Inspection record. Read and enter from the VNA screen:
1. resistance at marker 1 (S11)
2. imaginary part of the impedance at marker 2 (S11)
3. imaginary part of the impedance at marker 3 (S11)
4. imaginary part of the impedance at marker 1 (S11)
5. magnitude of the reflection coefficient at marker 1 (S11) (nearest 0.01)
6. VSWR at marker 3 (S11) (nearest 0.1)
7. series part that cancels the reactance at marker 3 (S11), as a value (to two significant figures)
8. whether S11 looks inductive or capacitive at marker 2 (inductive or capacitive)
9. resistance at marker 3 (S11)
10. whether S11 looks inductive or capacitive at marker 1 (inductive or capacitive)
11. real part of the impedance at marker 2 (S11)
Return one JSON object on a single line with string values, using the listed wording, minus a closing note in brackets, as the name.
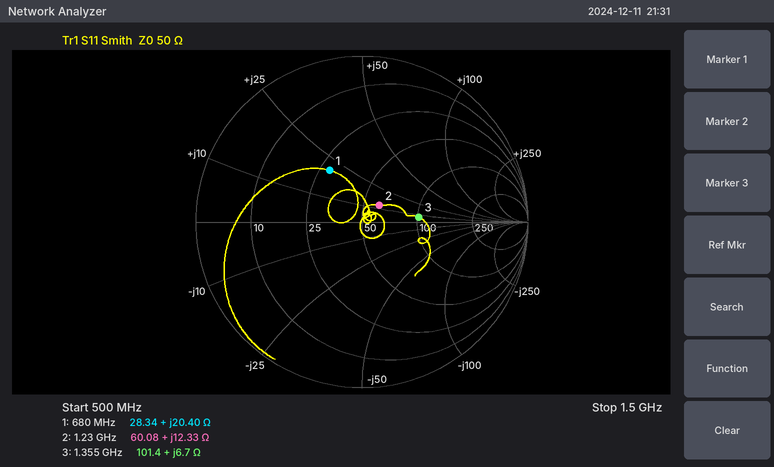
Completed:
{"resistance at marker 1": "28.34 Ω", "imaginary part of the impedance at marker 2": "+12.33 Ω", "imaginary part of the impedance at marker 3": "+6.7 Ω", "imaginary part of the impedance at marker 1": "+20.40 Ω", "magnitude of the reflection coefficient at marker 1 (S11)": "0.37", "VSWR at marker 3 (S11)": "2.0", "series part that cancels the reactance at marker 3 (S11), as a value": "18 pF", "whether S11 looks inductive or capacitive at marker 2": "inductive", "resistance at marker 3": "101.4 Ω", "whether S11 looks inductive or capacitive at marker 1": "inductive", "real part of the impedance at marker 2": "60.08 Ω"}
